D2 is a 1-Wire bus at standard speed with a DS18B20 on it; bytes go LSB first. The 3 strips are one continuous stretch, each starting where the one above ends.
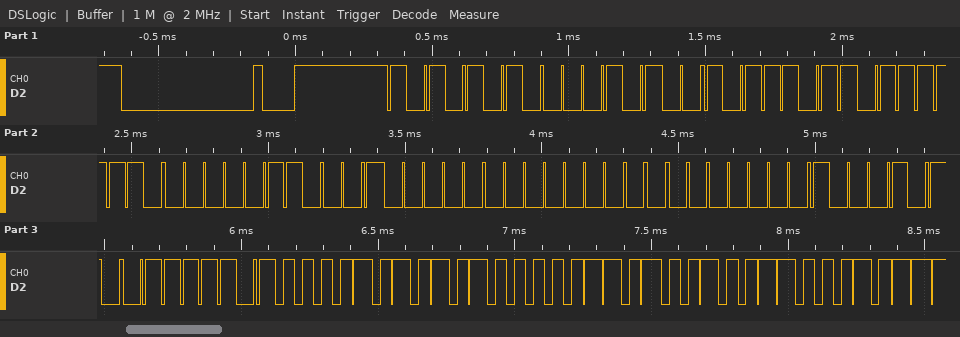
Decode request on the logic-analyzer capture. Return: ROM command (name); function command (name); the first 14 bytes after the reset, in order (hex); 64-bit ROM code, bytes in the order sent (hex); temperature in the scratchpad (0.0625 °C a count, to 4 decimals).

Match ROM
Read Scratchpad
55 28 DD 7E 60 04 00 00 51 BE 50 05 4B 46
28 DD 7E 60 04 00 00 51
85.0000 °C
